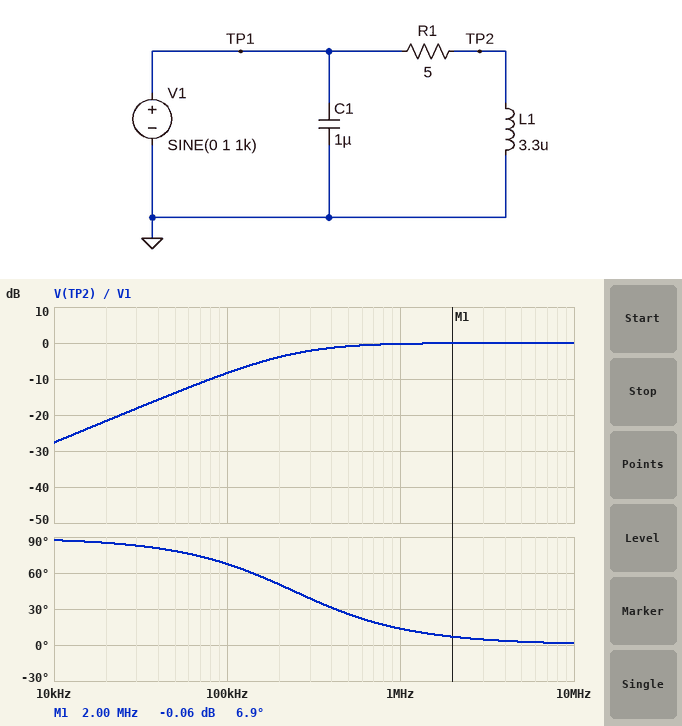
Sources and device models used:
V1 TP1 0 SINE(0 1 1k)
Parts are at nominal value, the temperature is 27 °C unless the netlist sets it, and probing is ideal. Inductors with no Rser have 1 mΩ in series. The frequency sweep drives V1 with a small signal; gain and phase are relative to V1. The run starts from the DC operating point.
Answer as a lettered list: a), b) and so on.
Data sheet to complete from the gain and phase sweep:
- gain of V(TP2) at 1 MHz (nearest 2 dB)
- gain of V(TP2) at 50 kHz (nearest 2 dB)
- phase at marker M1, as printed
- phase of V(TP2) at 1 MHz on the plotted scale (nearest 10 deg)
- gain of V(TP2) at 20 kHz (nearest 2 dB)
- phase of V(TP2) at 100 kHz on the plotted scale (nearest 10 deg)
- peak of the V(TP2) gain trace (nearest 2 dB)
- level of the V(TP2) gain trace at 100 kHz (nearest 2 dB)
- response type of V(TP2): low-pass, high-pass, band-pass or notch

a) 0 dB
b) -14 dB
c) 6.9 deg
d) 10 deg
e) -22 dB
f) 70 deg
g) 0 dB
h) -8 dB
i) high-pass
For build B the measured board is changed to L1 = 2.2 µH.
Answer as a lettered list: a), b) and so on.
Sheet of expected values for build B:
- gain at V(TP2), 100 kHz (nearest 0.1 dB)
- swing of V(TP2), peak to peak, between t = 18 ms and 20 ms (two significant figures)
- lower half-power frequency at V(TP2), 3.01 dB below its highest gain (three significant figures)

a) -11.5 dB
b) 5.5 mV
c) 362 kHz
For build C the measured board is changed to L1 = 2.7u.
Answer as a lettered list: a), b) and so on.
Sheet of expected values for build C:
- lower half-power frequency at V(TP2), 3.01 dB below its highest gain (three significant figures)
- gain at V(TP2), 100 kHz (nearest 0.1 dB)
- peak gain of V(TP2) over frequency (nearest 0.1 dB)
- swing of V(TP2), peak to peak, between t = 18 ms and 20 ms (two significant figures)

a) 295 kHz
b) -9.9 dB
c) 0 dB
d) 6.8 mV
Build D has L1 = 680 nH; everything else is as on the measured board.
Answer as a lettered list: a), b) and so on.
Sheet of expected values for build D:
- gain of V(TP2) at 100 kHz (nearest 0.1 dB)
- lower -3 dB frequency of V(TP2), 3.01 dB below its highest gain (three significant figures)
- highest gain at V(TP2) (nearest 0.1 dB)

a) -21.4 dB
b) 1.17 MHz
c) 0 dB
